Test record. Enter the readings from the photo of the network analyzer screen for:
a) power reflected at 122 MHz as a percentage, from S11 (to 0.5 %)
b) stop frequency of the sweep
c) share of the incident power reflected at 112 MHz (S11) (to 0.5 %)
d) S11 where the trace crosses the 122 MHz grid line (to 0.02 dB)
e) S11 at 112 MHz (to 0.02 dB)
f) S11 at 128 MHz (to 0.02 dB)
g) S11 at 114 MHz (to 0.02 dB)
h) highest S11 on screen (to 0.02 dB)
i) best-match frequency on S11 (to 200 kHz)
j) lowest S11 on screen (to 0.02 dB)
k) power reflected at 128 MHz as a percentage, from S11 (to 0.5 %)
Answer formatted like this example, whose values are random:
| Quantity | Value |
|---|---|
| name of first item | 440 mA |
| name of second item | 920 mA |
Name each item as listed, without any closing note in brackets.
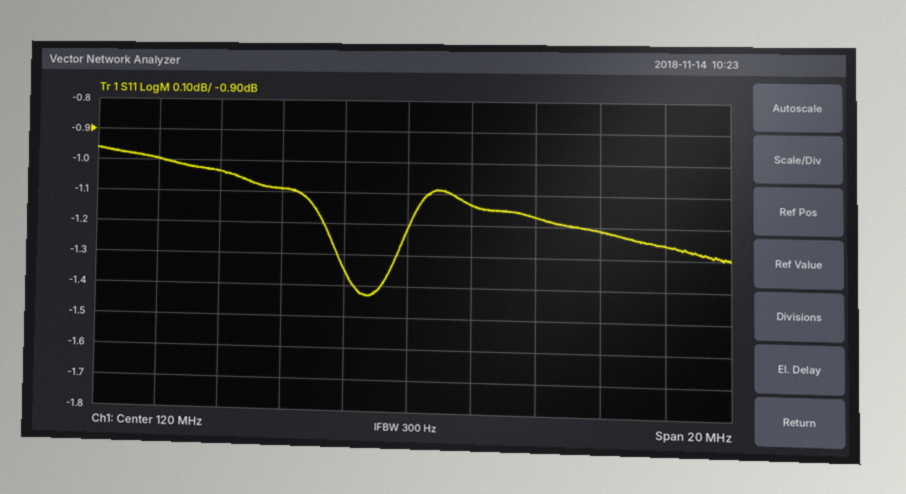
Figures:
| Quantity | Value |
|---|---|
| power reflected at 122 MHz as a percentage, from S11 | 77.0 % |
| stop frequency of the sweep | 130 MHz |
| share of the incident power reflected at 112 MHz (S11) | 79.5 % |
| S11 where the trace crosses the 122 MHz grid line | -1.14 dB |
| S11 at 112 MHz | -1.00 dB |
| S11 at 128 MHz | -1.26 dB |
| S11 at 114 MHz | -1.04 dB |
| highest S11 on screen | -0.96 dB |
| best-match frequency on S11 | 118.8 MHz |
| lowest S11 on screen | -1.44 dB |
| power reflected at 128 MHz as a percentage, from S11 | 75.0 % |
